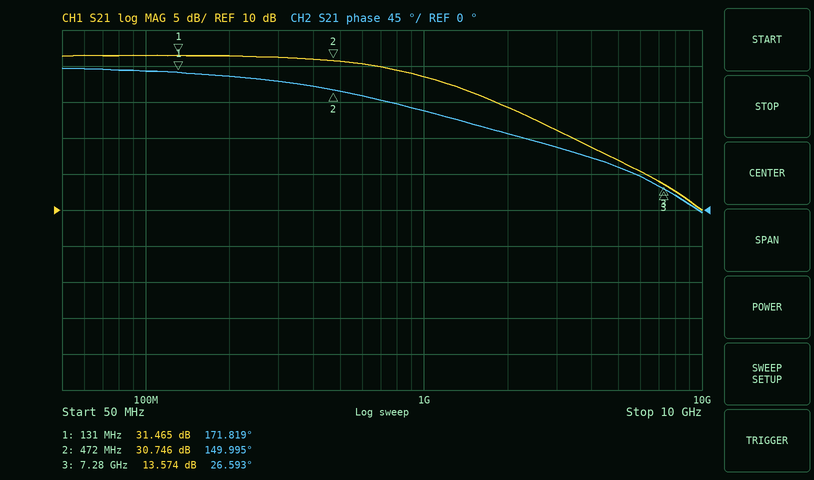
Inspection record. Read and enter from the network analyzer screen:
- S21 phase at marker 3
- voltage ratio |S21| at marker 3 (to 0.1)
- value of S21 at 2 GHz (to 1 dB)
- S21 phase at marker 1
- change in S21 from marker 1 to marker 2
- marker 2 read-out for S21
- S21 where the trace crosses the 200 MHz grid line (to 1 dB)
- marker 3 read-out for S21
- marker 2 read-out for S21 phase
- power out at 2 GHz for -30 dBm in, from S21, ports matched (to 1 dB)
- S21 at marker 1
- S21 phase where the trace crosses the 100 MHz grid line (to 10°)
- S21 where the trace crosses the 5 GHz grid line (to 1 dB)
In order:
26.593°
4.8
24 dB
171.819°
-0.719 dB
30.746 dB
31 dB
13.574 dB
149.995°
-6 dBm
31.465 dB
170°
17 dB
